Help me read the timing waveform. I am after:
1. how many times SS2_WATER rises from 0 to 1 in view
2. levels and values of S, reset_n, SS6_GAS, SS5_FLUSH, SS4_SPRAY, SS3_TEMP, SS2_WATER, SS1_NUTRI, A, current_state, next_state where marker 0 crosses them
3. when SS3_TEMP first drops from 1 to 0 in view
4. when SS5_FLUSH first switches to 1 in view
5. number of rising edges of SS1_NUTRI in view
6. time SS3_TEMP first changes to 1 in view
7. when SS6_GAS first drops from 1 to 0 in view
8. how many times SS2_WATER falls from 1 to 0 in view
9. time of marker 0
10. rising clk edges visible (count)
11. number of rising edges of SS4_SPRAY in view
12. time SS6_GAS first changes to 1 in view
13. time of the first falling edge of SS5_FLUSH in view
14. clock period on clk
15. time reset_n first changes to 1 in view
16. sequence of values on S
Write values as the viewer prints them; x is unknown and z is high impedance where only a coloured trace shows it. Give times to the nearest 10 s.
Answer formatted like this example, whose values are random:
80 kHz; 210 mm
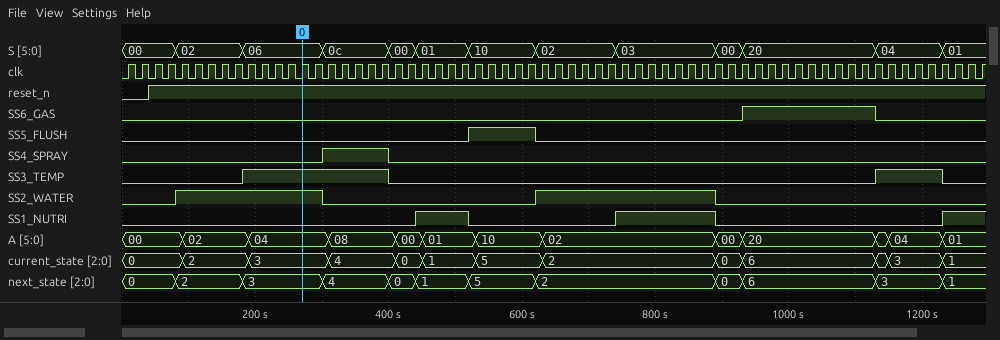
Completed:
2; S=06, reset_n=1, SS6_GAS=0, SS5_FLUSH=0, SS4_SPRAY=0, SS3_TEMP=1, SS2_WATER=1, SS1_NUTRI=0, A=04, current_state=3, next_state=3; 400 s; 520 s; 3; 180 s; 1130 s; 2; 270 s; 65; 1; 930 s; 620 s; 20 s; 40 s; 00, 02, 06, 0c, 00, 01, 10, 02, 03, 00, 20, 04, 01
